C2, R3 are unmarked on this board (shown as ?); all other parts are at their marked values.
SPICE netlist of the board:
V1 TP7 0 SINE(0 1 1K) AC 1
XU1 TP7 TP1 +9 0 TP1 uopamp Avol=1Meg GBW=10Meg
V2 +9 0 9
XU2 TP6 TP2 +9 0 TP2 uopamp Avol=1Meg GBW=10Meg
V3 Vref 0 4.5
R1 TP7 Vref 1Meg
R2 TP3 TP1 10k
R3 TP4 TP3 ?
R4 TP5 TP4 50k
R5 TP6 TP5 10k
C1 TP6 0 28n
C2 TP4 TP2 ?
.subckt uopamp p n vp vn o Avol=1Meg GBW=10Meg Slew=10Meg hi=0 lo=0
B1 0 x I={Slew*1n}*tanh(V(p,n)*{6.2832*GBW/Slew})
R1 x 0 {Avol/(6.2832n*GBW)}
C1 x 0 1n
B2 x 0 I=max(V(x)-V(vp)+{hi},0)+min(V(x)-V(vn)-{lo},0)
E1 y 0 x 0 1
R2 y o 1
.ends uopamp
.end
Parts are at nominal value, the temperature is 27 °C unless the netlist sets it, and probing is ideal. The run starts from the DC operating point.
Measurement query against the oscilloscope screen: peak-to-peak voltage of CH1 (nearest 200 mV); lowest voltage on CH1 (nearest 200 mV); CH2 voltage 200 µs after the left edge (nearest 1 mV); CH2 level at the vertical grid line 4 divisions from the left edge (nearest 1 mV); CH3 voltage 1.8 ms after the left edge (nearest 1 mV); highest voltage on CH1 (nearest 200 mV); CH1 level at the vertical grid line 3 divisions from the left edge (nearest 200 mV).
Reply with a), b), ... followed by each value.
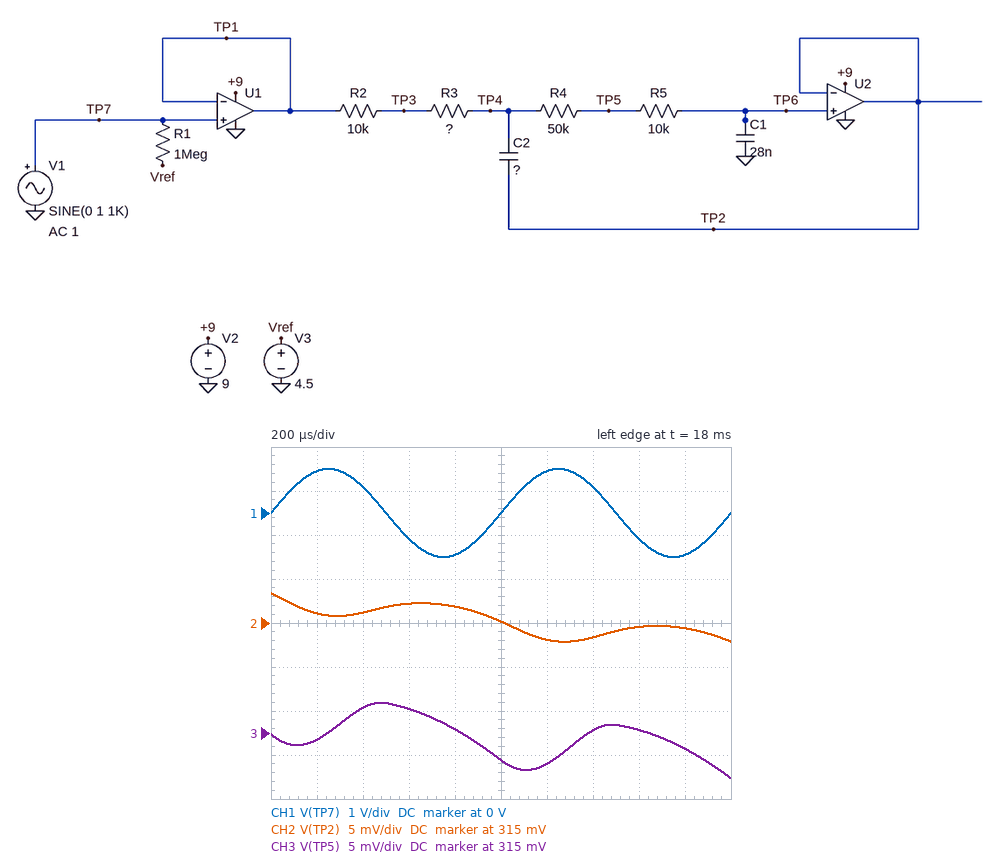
a) 2.0 V
b) -1.0 V
c) 316 mV
d) 317 mV
e) 313 mV
f) 1.0 V
g) -600 mV
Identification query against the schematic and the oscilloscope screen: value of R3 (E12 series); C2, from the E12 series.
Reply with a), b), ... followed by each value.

a) 56 kΩ
b) 82 nF
